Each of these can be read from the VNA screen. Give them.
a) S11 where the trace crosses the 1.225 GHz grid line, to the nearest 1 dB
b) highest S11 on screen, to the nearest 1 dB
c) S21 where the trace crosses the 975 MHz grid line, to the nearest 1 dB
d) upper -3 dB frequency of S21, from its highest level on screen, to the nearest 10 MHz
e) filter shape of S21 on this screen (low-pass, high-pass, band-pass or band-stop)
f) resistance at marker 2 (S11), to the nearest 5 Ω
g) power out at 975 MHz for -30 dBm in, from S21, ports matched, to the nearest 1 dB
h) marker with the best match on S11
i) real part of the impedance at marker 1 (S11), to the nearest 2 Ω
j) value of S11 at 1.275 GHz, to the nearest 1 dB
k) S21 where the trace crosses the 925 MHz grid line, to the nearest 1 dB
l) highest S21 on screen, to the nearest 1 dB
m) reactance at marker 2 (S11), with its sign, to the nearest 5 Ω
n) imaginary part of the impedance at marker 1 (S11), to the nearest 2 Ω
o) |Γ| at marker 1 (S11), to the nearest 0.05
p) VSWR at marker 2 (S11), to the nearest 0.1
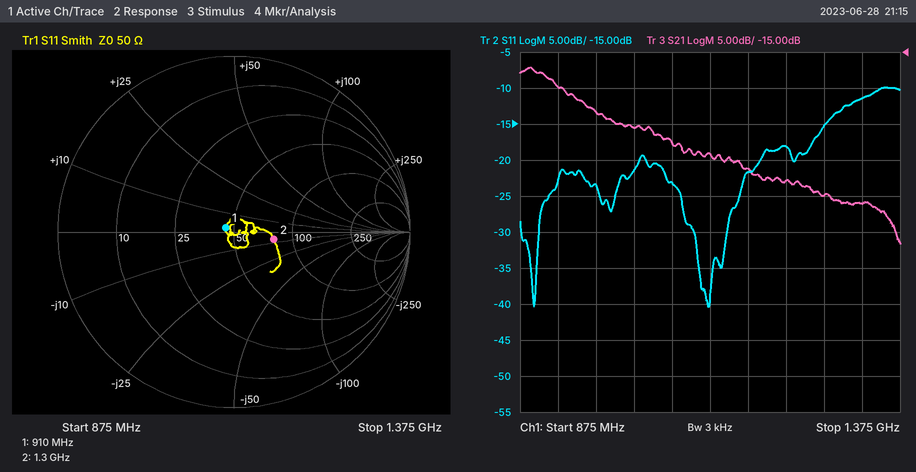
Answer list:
-18 dB
-10 dB
-23 dB
930 MHz
low-pass
80 Ω
-53 dBm
marker 1
46 Ω
-15 dB
-20 dB
-17 dB
-5 Ω
+2 Ω
0.05
1.6
